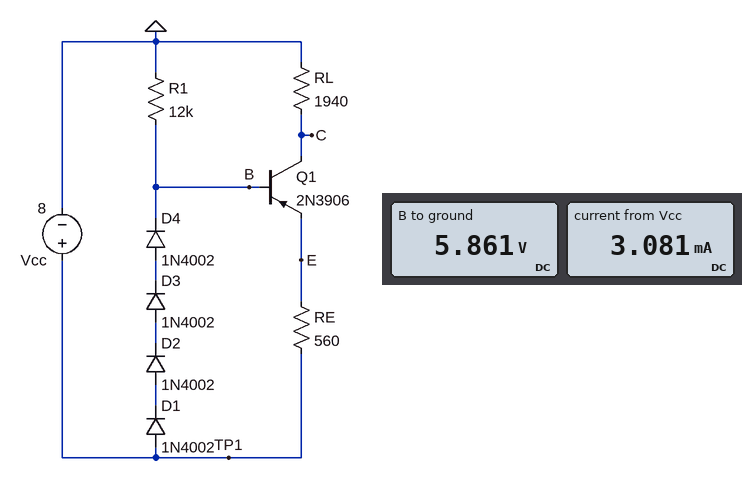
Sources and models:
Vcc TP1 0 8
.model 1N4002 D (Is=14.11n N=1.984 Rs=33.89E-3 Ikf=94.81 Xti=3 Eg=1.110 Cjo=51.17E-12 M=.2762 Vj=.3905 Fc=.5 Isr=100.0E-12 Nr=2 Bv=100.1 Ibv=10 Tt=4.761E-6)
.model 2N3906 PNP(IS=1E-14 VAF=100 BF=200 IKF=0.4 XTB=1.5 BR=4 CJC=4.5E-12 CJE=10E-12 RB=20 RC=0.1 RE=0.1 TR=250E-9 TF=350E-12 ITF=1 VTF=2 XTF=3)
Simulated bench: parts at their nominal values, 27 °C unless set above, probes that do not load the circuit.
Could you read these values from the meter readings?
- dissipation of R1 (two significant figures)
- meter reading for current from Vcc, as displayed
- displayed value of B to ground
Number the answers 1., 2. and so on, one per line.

1. 2.9 mW
2. 3.081 mA
3. 5.861 V
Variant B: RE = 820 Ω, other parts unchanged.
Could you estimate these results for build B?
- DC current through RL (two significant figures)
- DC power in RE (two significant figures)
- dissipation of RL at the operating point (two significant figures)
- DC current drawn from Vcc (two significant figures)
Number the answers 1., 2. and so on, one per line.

1. 1.8 mA
2. 2.6 mW
3. 6.2 mW
4. 2.3 mA
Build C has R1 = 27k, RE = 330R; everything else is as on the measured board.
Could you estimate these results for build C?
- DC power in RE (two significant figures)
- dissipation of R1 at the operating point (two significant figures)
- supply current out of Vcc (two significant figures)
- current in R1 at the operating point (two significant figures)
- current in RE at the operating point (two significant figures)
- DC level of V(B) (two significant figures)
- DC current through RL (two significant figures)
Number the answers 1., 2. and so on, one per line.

1. 4.2 mW
2. 1.4 mW
3. 3.7 mA
4. 230 µA
5. 3.6 mA
6. 6.1 V
7. 3.5 mA
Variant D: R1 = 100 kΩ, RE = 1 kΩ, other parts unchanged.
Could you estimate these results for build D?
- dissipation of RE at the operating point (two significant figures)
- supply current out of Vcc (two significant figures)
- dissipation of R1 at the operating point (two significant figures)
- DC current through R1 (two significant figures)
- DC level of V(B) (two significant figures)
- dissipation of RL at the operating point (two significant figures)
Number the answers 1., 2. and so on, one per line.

1. 1.1 mW
2. 1.1 mA
3. 400 µW
4. 63 µA
5. 6.3 V
6. 2.1 mW
